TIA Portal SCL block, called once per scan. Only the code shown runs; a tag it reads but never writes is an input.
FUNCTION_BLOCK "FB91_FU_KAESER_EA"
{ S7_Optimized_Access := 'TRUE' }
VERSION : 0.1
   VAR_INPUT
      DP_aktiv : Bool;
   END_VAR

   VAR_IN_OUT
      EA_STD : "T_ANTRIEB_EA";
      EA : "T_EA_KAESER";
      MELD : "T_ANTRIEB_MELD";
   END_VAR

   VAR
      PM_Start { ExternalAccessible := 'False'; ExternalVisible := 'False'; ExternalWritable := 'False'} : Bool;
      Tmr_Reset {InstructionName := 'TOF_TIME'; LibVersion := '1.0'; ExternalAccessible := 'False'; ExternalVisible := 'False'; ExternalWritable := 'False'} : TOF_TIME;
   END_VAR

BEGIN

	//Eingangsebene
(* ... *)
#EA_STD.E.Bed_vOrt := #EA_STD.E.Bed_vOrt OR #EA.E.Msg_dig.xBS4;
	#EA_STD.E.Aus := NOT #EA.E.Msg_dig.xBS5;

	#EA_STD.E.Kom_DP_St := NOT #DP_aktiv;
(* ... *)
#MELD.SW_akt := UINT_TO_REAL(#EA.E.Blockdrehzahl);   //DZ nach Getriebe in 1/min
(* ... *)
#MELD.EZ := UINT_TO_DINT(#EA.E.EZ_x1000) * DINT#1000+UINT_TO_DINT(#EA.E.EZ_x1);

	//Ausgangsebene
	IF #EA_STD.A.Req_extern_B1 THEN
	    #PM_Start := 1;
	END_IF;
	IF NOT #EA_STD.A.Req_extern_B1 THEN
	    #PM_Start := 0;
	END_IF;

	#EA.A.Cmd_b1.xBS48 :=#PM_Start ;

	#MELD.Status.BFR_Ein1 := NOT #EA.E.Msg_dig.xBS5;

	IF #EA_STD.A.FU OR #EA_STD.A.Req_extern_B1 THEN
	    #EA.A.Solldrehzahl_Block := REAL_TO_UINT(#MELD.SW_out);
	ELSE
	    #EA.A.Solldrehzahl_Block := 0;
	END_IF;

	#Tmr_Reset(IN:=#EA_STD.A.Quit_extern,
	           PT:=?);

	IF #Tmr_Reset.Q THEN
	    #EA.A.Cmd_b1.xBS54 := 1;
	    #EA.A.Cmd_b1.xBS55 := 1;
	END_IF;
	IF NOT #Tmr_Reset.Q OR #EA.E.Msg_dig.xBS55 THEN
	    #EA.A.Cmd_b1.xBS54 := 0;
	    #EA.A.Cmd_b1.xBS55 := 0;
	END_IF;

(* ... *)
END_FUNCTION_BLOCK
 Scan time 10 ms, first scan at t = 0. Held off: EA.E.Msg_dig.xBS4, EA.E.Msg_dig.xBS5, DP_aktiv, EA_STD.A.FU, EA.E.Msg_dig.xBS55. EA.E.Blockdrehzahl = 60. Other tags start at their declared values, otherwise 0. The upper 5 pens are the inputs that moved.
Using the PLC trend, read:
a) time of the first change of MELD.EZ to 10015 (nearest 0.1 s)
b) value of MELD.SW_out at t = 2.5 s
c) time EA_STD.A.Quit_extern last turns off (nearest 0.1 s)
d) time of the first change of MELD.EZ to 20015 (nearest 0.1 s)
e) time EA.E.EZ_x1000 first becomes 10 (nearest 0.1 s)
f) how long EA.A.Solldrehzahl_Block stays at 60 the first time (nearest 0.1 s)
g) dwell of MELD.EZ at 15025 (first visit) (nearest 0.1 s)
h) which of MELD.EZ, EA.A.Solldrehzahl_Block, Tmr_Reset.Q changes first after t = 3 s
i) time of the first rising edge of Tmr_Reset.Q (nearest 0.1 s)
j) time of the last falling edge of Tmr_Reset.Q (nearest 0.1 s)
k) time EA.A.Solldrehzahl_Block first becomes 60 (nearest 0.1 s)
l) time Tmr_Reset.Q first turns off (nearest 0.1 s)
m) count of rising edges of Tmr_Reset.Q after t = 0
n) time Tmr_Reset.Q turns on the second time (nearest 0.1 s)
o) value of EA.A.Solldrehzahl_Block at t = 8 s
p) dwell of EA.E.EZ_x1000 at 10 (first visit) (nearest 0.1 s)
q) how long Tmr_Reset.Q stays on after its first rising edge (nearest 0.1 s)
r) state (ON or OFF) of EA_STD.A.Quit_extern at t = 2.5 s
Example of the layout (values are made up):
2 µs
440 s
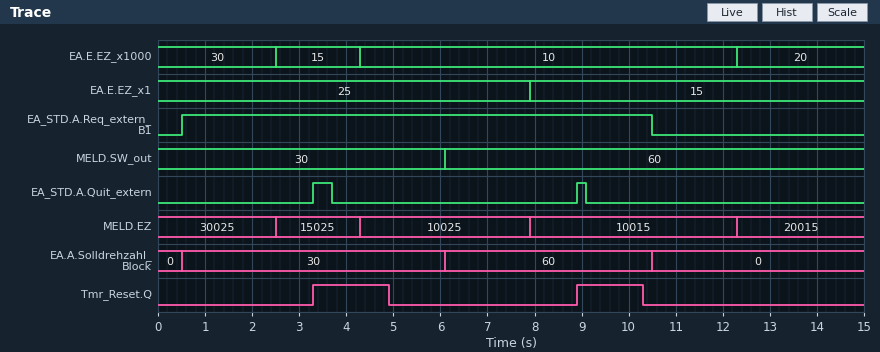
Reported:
7.9 s
30
9.1 s
12.3 s
4.3 s
4.4 s
1.8 s
Tmr_Reset.Q
3.3 s
10.3 s
6.1 s
4.9 s
2
8.9 s
60
8.0 s
1.6 s
OFF
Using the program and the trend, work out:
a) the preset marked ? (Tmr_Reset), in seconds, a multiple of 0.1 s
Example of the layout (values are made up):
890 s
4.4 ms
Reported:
1.2 s
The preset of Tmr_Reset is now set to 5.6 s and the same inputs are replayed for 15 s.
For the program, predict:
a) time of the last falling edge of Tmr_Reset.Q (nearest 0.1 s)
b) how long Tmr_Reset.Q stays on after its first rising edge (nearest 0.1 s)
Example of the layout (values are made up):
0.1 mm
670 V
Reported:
14.7 s
11.4 s
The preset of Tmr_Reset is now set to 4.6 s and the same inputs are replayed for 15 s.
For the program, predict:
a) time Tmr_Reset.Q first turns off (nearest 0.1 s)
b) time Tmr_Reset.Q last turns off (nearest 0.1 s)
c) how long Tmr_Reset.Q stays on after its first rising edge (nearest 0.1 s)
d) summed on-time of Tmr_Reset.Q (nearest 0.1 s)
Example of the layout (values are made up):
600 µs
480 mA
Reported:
8.3 s
13.7 s
5.0 s
9.8 s
